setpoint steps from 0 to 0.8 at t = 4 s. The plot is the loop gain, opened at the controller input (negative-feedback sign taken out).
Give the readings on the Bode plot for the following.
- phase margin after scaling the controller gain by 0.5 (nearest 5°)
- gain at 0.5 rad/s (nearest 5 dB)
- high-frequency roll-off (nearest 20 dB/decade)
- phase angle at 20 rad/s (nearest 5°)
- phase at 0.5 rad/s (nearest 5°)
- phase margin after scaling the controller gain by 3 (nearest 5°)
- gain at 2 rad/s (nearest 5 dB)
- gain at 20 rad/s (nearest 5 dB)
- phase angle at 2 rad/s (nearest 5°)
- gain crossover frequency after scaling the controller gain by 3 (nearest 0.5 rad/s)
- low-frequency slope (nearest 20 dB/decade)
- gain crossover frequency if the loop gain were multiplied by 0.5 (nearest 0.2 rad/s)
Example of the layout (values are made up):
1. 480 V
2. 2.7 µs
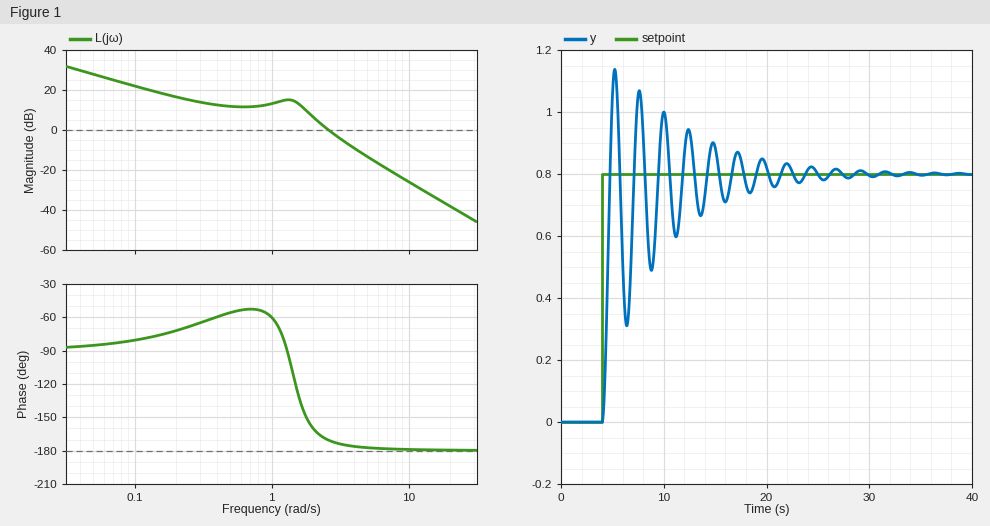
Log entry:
1. 20°
2. 10 dB
3. -40 dB/decade
4. -180°
5. -55°
6. 5°
7. 5 dB
8. -40 dB
9. -160°
10. 4.0 rad/s
11. -20 dB/decade
12. 2.0 rad/s
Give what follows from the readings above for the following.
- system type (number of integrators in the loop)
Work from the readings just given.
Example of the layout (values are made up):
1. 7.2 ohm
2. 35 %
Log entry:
1. 1
